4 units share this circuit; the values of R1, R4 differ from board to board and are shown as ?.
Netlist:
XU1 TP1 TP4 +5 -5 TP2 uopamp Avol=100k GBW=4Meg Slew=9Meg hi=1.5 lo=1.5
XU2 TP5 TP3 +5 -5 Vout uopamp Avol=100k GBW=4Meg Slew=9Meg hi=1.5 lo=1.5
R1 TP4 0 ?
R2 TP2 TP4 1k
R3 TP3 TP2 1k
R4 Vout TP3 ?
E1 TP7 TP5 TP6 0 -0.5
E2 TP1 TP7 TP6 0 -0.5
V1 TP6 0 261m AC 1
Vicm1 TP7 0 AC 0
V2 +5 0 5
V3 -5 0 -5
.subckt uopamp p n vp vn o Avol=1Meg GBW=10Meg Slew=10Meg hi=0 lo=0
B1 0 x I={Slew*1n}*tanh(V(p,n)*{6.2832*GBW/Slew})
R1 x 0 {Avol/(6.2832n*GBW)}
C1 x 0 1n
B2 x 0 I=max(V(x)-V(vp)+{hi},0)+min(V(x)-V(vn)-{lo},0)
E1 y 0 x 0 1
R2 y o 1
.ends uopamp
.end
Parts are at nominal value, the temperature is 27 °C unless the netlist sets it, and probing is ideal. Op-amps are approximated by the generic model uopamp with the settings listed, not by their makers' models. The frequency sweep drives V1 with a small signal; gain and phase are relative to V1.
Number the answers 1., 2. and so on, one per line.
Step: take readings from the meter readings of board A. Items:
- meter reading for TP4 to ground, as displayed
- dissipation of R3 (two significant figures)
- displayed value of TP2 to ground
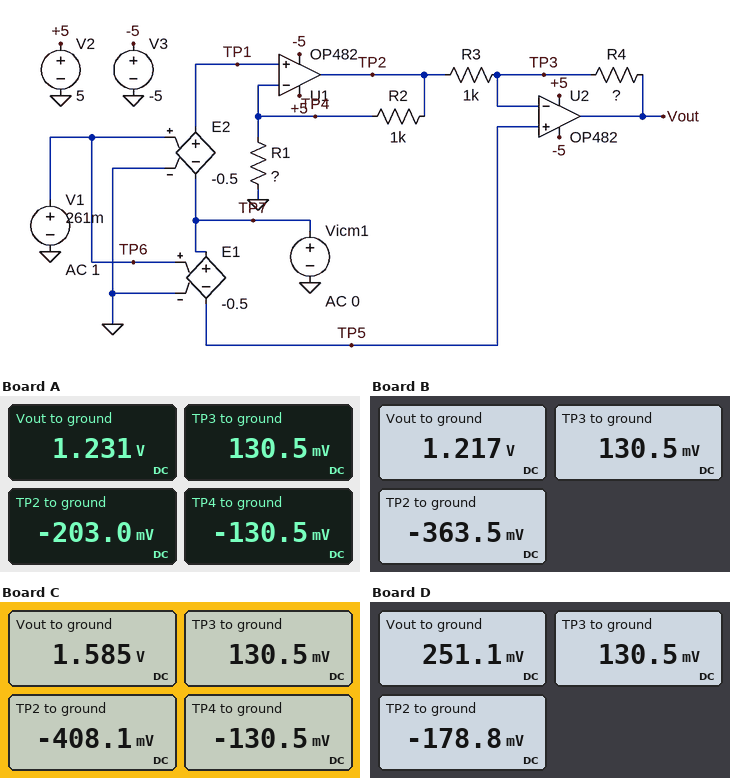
1. -130.5 mV
2. 110 µW
3. -203.0 mV
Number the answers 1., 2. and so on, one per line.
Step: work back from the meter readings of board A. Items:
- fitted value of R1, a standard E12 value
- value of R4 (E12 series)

1. 1.8 kΩ
2. 3.3 kΩ
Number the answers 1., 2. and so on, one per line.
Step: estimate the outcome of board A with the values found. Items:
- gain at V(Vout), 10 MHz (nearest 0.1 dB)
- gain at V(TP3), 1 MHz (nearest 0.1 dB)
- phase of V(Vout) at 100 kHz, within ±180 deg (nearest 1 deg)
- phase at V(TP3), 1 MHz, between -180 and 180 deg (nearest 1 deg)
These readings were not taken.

1. -13.1 dB
2. -7.4 dB
3. -7 deg
4. -110 deg
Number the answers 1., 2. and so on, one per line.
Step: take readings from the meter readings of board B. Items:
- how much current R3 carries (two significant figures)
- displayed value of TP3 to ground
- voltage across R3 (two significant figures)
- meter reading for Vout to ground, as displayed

1. 490 µA
2. 130.5 mV
3. 490 mV
4. 1.217 V
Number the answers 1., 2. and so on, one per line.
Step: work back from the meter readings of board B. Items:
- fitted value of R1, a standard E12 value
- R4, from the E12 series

1. 560 Ω
2. 2.2 kΩ
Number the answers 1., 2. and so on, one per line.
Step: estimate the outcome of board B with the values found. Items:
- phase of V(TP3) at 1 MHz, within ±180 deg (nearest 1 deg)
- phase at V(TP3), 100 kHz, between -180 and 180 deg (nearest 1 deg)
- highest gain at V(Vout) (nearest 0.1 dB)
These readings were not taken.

1. -113 deg
2. -13 deg
3. 13.4 dB
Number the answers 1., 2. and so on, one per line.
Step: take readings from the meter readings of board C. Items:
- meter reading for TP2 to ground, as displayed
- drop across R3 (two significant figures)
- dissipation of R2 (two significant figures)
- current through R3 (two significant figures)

1. -408.1 mV
2. 540 mV
3. 77 µW
4. 540 µA
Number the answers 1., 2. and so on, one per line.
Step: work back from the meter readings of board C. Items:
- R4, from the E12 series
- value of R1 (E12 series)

1. 2.7 kΩ
2. 470 Ω
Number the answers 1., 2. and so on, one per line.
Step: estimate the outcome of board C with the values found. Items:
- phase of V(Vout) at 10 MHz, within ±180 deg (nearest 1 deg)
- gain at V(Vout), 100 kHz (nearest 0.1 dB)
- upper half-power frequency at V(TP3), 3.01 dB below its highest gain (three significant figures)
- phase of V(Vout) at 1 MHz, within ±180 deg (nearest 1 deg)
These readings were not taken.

1. -99 deg
2. 15.6 dB
3. 2.04 MHz
4. -67 deg
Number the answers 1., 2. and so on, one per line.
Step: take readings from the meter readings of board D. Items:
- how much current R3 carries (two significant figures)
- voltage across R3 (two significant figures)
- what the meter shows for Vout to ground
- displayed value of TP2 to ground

1. 310 µA
2. 310 mV
3. 251.1 mV
4. -178.8 mV
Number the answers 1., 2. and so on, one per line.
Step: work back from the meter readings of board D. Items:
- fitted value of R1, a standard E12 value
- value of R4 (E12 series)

1. 2.7 kΩ
2. 390 Ω
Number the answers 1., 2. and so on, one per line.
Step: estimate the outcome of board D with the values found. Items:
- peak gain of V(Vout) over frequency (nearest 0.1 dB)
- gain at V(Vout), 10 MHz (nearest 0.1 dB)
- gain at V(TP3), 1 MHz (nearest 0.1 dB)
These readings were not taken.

1. -0.3 dB
2. -14.0 dB
3. -6.8 dB
